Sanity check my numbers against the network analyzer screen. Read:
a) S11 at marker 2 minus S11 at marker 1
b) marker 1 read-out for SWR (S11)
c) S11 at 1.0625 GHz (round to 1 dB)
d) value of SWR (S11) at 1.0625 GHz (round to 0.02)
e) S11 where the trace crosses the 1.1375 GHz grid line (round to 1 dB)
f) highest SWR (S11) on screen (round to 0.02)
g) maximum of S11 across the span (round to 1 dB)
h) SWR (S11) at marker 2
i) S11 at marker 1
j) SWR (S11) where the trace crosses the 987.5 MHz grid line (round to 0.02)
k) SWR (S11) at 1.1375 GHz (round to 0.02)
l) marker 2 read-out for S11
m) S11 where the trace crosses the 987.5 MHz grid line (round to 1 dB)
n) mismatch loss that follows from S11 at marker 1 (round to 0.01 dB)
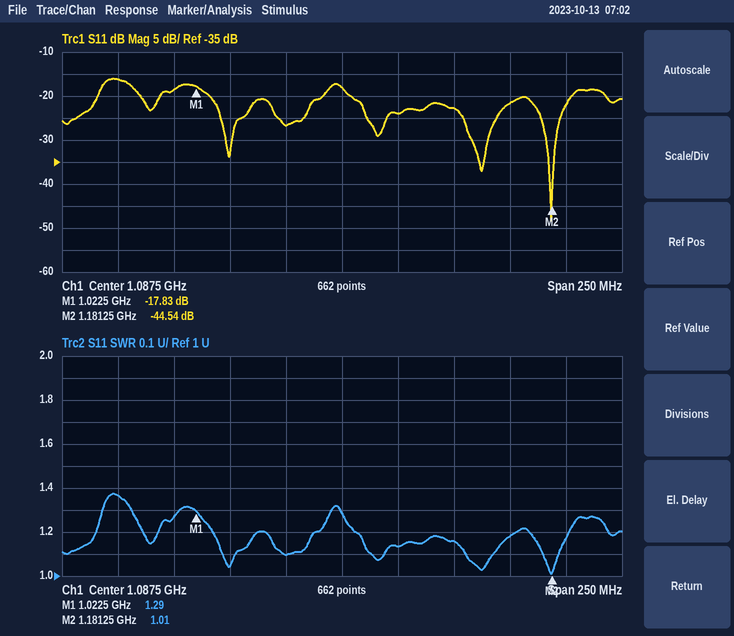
-26.71 dB
1.29
-27 dB
1.10
-23 dB
1.38
-16 dB
1.01
-17.83 dB
1.36
1.16
-44.54 dB
-16 dB
0.07 dB
